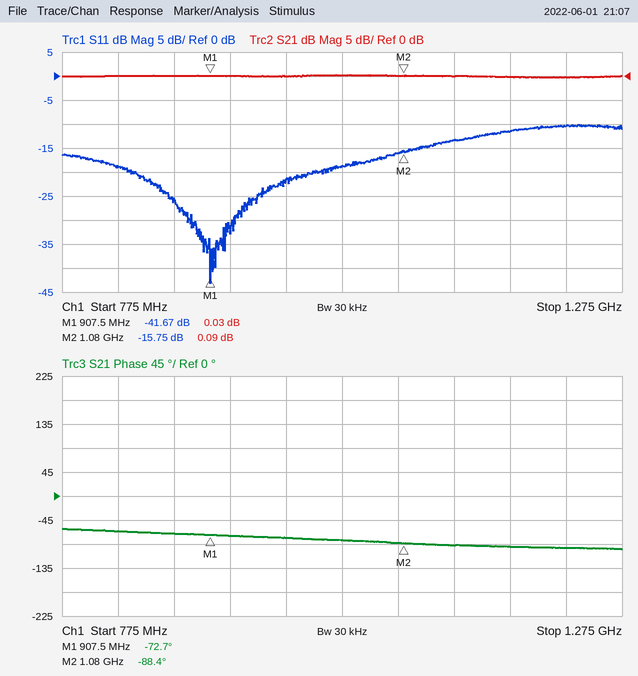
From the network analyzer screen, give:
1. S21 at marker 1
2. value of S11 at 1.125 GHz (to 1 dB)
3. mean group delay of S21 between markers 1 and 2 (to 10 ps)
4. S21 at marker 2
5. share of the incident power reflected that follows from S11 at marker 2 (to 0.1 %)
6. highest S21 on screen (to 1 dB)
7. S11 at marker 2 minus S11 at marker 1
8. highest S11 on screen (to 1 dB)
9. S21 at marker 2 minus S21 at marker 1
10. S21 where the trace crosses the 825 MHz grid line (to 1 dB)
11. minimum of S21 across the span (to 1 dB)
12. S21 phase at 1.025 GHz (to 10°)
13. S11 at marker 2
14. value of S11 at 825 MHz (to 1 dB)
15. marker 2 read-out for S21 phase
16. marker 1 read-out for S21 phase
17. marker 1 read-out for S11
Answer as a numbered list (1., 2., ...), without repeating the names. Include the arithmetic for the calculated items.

1. 0.03 dB
2. -13 dB
3. −(-88.4° − (-72.7°))/(360° × 172.5 MHz) ≈ 253 ps, so 250 ps to the nearest 10 ps
4. 0.09 dB
5. 10^(-15.75/10) ≈ 2.7 %
6. 0 dB
7. -15.75 − (-41.67) = 25.92 dB
8. -10 dB
9. 0.09 − (0.03) = 0.06 dB
10. 0 dB
11. 0 dB
12. -80°
13. -15.75 dB
14. -19 dB
15. -88.4°
16. -72.7°
17. -41.67 dB
